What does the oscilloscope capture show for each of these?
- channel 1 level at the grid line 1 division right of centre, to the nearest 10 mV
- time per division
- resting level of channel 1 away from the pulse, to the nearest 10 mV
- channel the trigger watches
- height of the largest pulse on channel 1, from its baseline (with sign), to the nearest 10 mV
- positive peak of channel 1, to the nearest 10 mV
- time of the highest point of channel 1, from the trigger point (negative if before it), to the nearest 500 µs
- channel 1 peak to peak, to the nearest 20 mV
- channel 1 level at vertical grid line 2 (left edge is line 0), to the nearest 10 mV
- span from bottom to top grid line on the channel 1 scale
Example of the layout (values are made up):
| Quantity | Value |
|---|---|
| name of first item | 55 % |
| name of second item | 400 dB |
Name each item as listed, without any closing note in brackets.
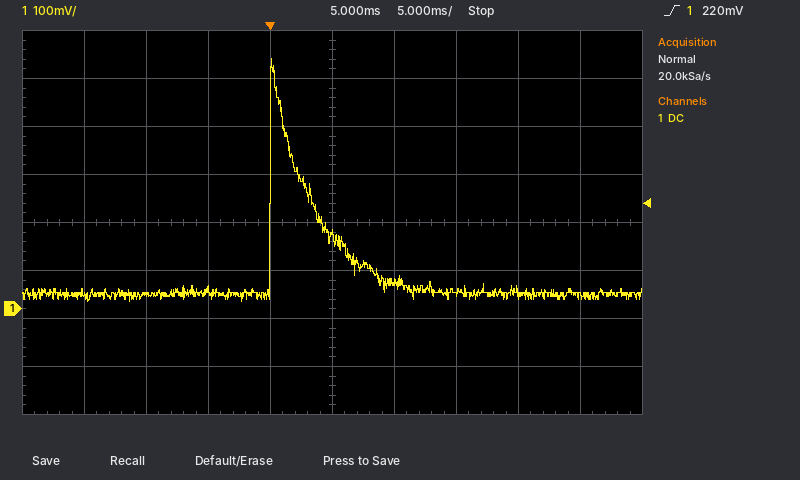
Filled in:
| Quantity | Value |
|---|---|
| channel 1 level at the grid line 1 division right of centre, to the nearest 10 mV | 60 mV |
| time per division | 5 ms |
| resting level of channel 1 away from the pulse, to the nearest 10 mV | 30 mV |
| channel the trigger watches | channel 1 |
| height of the largest pulse on channel 1, from its baseline (with sign), to the nearest 10 mV | +490 mV |
| positive peak of channel 1, to the nearest 10 mV | 520 mV |
| time of the highest point of channel 1, from the trigger point (negative if before it), to the nearest 500 µs | 0.0 ms |
| channel 1 peak to peak, to the nearest 20 mV | 500 mV |
| channel 1 level at vertical grid line 2 (left edge is line 0), to the nearest 10 mV | 30 mV |
| span from bottom to top grid line on the channel 1 scale | 800 mV |
